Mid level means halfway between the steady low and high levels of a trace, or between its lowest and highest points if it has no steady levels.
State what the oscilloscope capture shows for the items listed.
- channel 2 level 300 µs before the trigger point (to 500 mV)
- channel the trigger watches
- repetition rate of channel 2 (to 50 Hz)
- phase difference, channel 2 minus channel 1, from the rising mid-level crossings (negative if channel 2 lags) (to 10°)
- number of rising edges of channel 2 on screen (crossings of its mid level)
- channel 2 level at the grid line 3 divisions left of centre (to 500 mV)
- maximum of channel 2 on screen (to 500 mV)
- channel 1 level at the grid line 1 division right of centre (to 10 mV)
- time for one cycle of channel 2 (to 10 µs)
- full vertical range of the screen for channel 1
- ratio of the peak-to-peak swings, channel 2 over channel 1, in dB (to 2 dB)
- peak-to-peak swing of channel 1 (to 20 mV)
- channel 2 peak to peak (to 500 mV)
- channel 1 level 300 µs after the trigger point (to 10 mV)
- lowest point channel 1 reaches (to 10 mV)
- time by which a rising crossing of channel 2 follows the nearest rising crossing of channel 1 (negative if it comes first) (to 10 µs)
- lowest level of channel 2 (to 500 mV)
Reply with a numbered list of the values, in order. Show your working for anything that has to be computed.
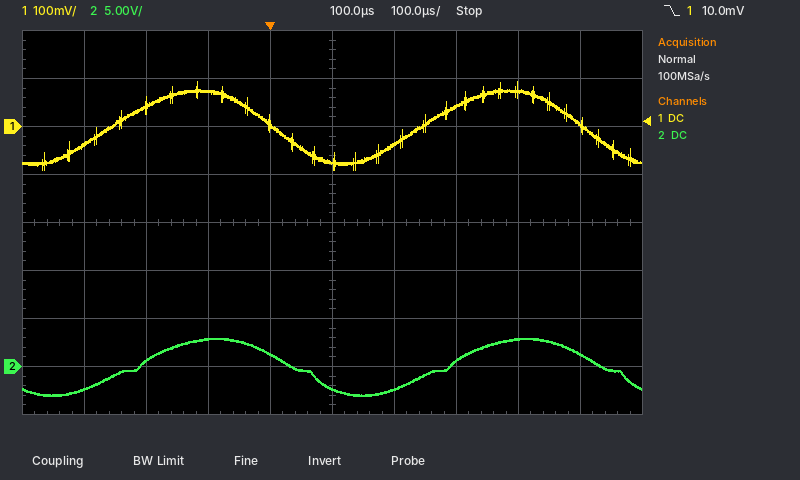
1. -2.5 V
2. channel 1
3. 1 / 500 µs ≈ 2.00 kHz
4. −360° × (+40 µs) / 500 µs ≈ -28.8°, so -30° to the nearest 10°
5. 2
6. 500 mV
7. 3.0 V
8. -40 mV
9. 500 µs
10. 800 mV
11. 20 log10(6.0 V / 180 mV) ≈ 30 dB
12. 180 mV
13. 3.0 V − (-3.0 V) = 6.0 V
14. 40 mV
15. -90 mV
16. +40 µs
17. -3.0 V
